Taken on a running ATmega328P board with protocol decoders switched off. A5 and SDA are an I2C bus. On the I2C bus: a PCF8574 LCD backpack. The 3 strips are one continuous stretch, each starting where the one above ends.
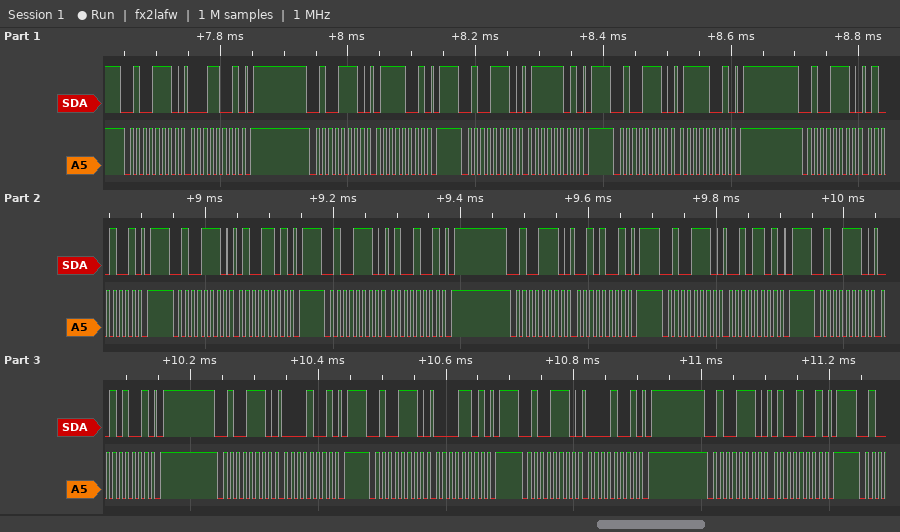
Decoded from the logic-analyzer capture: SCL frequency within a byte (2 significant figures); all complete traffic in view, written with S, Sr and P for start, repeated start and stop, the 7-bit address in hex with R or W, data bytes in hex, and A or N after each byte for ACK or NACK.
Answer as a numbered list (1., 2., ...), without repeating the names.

1. 100 kHz
2. S 27W A 19 A P S 27W A 79 A P S 27W A 7D A P S 27W A 79 A P S 27W A 49 A P S 27W A 4D A P S 27W A 49 A P S 27W A 29 A P S 27W A 2D A P S 27W A 29 A P S 27W A 09 A P S 27W A 0D A P S 27W A 09 A P S 27W A 49 A P
